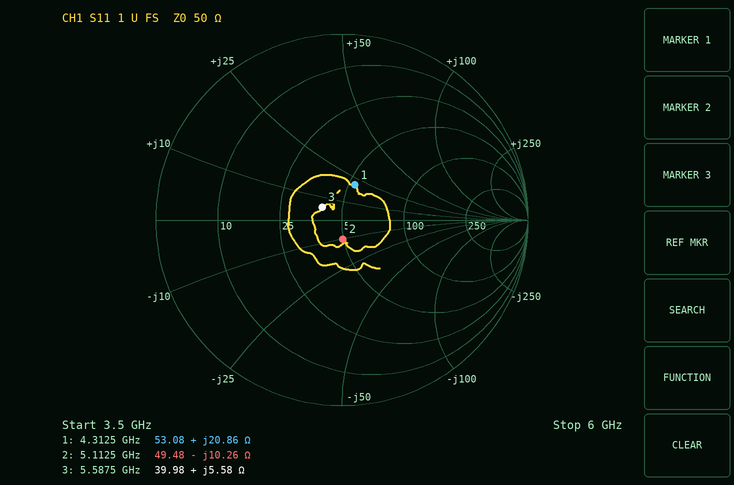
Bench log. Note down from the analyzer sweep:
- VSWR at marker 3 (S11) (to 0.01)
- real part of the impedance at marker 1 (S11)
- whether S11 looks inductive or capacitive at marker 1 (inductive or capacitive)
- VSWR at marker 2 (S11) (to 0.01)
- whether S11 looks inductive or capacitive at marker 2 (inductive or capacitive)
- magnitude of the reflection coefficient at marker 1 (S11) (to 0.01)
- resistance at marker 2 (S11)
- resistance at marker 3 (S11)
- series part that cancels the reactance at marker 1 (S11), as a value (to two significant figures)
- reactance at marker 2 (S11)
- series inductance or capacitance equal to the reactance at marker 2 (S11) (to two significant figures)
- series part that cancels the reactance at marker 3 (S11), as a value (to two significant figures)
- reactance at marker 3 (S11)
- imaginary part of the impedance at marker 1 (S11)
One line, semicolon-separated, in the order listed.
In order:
1.29; 53.08 Ω; inductive; 1.23; capacitive; 0.20; 49.48 Ω; 39.98 Ω; 1.8 pF; -10.26 Ω; 3.0 pF; 5.1 pF; +5.58 Ω; +20.86 Ω
